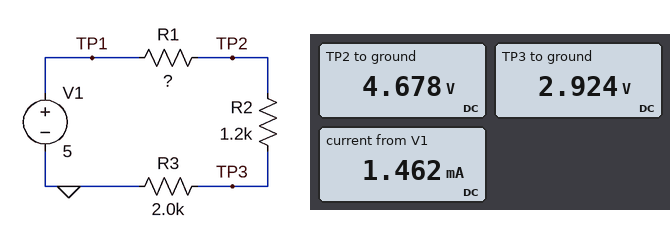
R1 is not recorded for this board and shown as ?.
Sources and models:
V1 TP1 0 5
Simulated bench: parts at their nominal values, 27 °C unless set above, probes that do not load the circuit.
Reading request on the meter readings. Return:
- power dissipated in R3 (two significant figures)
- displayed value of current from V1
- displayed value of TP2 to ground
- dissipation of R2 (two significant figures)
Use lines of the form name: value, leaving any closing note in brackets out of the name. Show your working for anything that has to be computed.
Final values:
power dissipated in R3: (2.924 V)^2 / 2 kΩ = 4.3 mW
displayed value of current from V1: 1.462 mA
displayed value of TP2 to ground: 4.678 V
dissipation of R2: (4.678 V - 2.924 V)^2 / 1.2 kΩ = 2.6 mW
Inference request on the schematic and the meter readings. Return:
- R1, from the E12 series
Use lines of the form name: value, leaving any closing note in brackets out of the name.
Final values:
R1, from the E12 series: 220 Ω
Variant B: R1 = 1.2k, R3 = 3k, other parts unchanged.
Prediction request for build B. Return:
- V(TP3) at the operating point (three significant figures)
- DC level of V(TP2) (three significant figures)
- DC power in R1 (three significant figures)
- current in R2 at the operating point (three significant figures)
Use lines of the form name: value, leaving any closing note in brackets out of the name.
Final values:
V(TP3) at the operating point: 2.78 V
DC level of V(TP2): 3.89 V
DC power in R1: 1.03 mW
current in R2 at the operating point: 926 µA
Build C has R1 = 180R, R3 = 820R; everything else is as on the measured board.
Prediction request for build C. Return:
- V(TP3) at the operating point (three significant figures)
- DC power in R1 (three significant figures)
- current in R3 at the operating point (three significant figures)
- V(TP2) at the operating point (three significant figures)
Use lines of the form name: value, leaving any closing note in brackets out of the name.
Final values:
V(TP3) at the operating point: 1.86 V
DC power in R1: 930 µW
current in R3 at the operating point: 2.27 mA
V(TP2) at the operating point: 4.59 V
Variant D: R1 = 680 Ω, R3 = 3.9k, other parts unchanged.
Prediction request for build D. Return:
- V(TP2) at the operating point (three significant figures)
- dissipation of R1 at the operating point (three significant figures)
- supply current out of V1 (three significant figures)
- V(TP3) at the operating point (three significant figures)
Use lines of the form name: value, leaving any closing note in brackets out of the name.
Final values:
V(TP2) at the operating point: 4.41 V
dissipation of R1 at the operating point: 509 µW
supply current out of V1: 865 µA
V(TP3) at the operating point: 3.37 V
